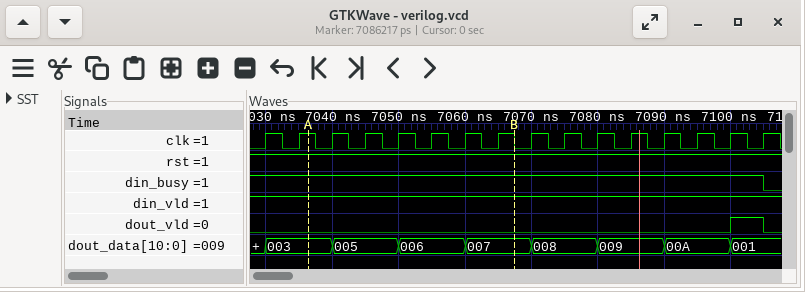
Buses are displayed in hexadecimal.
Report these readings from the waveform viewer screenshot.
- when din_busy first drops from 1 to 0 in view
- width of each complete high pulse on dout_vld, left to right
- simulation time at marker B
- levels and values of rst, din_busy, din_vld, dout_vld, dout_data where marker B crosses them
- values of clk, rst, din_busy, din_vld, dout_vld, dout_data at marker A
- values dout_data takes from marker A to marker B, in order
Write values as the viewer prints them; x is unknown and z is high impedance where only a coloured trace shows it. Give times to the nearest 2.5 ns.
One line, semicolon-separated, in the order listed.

7105 ns; 5 ns; 7067.5 ns; rst=1, din_busy=1, din_vld=1, dout_vld=0, dout_data=007; clk=1, rst=1, din_busy=1, din_vld=1, dout_vld=0, dout_data=003; 003, 005, 006, 007
